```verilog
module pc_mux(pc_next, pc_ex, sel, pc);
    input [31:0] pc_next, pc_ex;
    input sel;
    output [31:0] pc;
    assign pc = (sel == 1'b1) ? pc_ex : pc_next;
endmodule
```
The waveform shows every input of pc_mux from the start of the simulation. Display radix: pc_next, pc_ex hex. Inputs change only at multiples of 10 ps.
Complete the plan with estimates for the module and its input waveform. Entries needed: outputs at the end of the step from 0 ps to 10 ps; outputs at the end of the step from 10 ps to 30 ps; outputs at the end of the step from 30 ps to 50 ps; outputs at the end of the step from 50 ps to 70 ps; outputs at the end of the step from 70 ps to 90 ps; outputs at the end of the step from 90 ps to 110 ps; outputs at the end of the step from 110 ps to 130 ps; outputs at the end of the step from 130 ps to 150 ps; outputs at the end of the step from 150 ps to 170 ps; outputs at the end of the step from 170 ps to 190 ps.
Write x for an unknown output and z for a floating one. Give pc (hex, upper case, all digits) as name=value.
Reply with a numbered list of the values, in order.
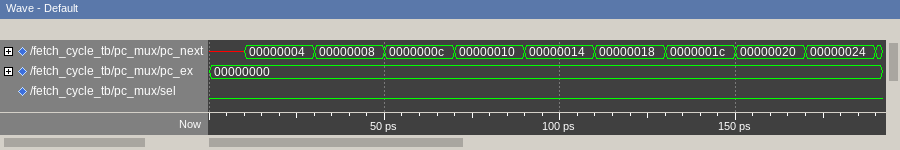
1. pc=x
2. pc=00000004
3. pc=00000008
4. pc=0000000C
5. pc=00000010
6. pc=00000014
7. pc=00000018
8. pc=0000001C
9. pc=00000020
10. pc=00000024
